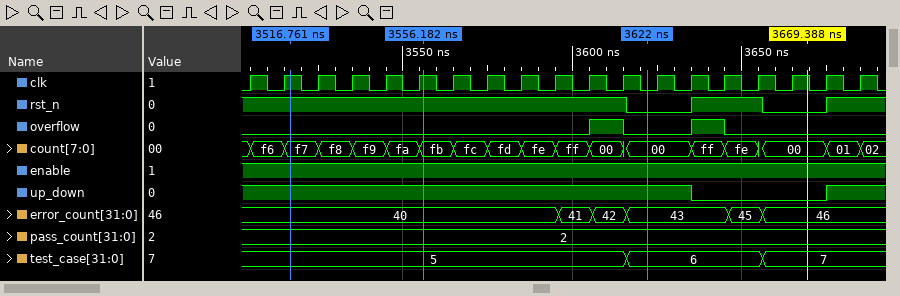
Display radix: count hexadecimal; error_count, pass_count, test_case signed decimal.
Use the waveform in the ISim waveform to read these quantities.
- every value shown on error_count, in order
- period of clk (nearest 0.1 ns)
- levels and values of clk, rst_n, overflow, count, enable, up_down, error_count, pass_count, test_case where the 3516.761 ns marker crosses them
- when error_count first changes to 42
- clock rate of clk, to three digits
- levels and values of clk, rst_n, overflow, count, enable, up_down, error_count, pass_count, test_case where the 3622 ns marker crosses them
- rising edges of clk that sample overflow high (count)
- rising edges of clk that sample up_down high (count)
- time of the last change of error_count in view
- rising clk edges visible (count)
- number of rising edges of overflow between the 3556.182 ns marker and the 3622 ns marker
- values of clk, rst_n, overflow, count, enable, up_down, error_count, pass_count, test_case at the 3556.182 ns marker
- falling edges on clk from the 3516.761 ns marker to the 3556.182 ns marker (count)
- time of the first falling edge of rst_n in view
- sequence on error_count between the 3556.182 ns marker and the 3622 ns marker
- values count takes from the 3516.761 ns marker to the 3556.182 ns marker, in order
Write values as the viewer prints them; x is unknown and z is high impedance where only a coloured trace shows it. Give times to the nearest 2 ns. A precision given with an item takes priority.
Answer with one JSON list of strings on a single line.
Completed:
["40, 41, 42, 43, 45, 46", "10 ns", "clk=1, rst_n=1, overflow=0, count=f7, enable=1, up_down=1, error_count=40, pass_count=2, test_case=5", "3606 ns", "100 MHz", "clk=0, rst_n=0, overflow=0, count=00, enable=1, up_down=1, error_count=43, pass_count=2, test_case=6", "2", "15", "3656 ns", "19", "1", "clk=1, rst_n=1, overflow=0, count=fb, enable=1, up_down=1, error_count=40, pass_count=2, test_case=5", "4", "3616 ns", "40, 41, 42, 43", "f7, f8, f9, fa, fb"]
